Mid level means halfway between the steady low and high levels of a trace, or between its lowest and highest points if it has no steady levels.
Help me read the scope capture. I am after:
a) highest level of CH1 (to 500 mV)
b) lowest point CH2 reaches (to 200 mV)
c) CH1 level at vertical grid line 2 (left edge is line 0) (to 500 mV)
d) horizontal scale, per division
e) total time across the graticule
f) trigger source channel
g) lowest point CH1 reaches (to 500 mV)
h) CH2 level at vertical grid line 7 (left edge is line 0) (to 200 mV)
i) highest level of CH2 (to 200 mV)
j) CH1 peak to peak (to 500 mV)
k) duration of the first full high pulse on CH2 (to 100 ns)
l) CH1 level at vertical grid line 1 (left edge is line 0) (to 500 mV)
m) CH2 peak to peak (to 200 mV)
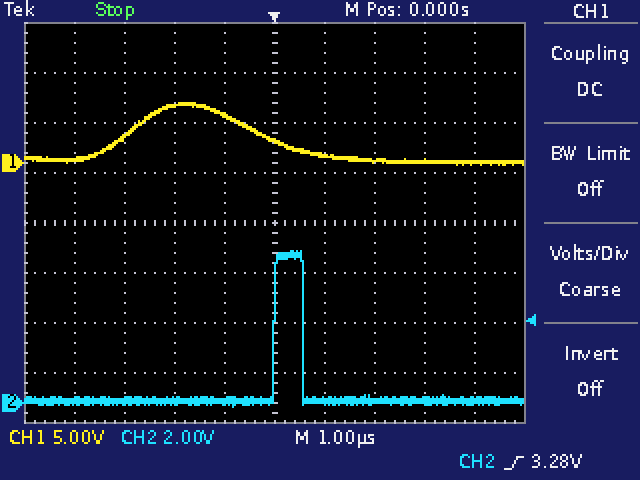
6.0 V
-200 mV
2.5 V
1 µs
10 µs
CH2
0.0 V
0.0 V
6.0 V
6.0 V
600 ns
500 mV
6.2 V
